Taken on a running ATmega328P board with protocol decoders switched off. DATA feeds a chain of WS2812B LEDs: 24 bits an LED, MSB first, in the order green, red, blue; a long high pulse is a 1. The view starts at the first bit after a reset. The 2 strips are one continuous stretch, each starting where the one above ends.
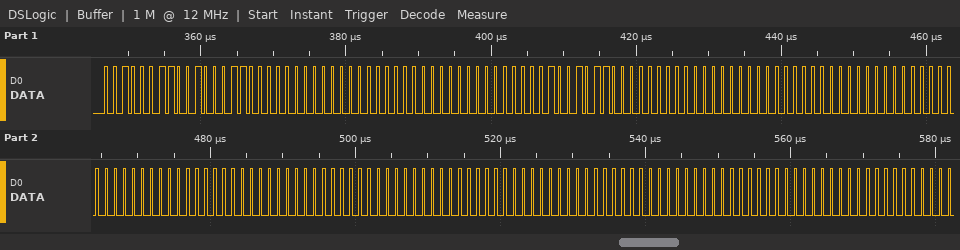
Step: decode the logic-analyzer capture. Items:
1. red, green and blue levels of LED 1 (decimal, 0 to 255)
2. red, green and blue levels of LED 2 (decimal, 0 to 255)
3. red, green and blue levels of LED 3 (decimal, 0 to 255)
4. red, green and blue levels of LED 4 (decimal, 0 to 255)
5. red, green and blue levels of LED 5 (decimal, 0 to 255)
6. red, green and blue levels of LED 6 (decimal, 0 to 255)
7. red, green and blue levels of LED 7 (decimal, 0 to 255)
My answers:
35, 35, 0
0, 0, 0
0, 75, 0
0, 0, 0
0, 0, 0
0, 0, 0
0, 0, 0
